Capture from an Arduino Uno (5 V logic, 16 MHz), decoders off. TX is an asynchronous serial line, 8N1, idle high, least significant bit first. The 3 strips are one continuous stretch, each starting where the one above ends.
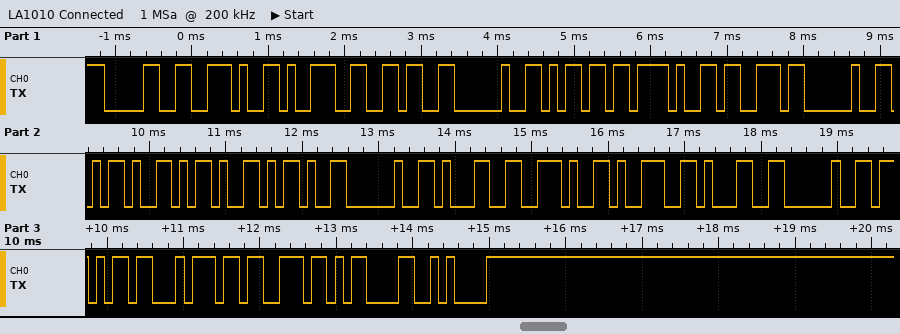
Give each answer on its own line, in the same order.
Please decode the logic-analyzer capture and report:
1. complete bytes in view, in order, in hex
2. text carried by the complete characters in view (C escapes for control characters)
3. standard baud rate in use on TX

30 2E 39 36 20 6D 2F 73 20 2D 2D 2D 20 31 2E 39 31 20 6B 74 73 0D 0A
"0.96 m/s --- 1.91 kts\r\n"
9600 baud
